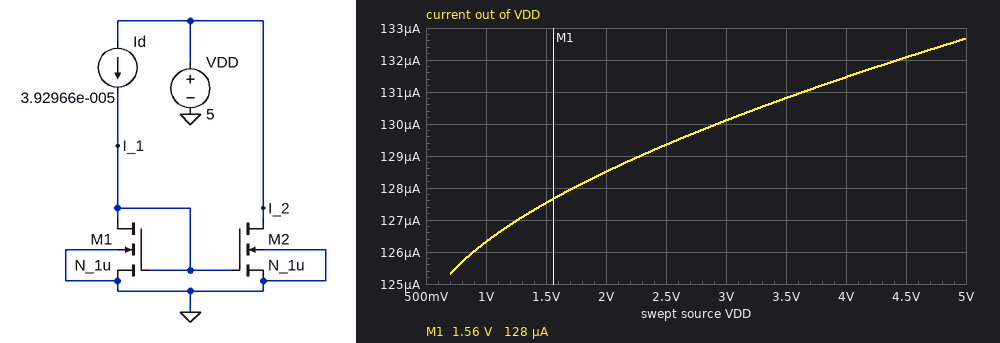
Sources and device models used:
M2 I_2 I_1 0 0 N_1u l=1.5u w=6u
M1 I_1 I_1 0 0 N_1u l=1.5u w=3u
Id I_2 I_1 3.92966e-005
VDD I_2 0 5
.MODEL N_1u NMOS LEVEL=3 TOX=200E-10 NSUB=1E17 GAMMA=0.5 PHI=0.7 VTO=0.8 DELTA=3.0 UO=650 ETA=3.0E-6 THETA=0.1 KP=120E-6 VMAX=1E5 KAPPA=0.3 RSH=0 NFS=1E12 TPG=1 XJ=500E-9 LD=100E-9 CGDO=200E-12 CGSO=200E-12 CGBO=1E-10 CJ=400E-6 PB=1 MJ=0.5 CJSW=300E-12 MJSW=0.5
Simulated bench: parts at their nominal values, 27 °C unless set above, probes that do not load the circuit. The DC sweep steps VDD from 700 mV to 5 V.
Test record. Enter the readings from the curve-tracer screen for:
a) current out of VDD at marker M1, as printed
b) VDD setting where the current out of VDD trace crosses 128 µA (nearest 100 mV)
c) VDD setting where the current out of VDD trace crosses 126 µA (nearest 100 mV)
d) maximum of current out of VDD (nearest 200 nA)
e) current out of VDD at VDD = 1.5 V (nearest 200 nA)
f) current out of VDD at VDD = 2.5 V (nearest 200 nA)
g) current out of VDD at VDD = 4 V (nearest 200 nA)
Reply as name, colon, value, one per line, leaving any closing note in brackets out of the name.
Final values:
current out of VDD at marker M1, as printed: 128 µA
VDD setting where the current out of VDD trace crosses 128 µA: 1.7 V
VDD setting where the current out of VDD trace crosses 126 µA: 900 mV
maximum of current out of VDD: 132.6 µA
current out of VDD at VDD = 1.5 V: 127.6 µA
current out of VDD at VDD = 2.5 V: 129.4 µA
current out of VDD at VDD = 4 V: 131.4 µA
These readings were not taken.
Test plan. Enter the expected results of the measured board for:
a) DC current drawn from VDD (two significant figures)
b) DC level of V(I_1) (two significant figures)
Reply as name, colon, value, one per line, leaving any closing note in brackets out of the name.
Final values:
DC current drawn from VDD: 130 µA
DC level of V(I_1): 1.5 V
